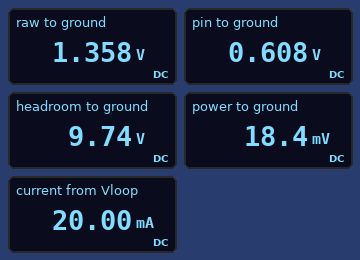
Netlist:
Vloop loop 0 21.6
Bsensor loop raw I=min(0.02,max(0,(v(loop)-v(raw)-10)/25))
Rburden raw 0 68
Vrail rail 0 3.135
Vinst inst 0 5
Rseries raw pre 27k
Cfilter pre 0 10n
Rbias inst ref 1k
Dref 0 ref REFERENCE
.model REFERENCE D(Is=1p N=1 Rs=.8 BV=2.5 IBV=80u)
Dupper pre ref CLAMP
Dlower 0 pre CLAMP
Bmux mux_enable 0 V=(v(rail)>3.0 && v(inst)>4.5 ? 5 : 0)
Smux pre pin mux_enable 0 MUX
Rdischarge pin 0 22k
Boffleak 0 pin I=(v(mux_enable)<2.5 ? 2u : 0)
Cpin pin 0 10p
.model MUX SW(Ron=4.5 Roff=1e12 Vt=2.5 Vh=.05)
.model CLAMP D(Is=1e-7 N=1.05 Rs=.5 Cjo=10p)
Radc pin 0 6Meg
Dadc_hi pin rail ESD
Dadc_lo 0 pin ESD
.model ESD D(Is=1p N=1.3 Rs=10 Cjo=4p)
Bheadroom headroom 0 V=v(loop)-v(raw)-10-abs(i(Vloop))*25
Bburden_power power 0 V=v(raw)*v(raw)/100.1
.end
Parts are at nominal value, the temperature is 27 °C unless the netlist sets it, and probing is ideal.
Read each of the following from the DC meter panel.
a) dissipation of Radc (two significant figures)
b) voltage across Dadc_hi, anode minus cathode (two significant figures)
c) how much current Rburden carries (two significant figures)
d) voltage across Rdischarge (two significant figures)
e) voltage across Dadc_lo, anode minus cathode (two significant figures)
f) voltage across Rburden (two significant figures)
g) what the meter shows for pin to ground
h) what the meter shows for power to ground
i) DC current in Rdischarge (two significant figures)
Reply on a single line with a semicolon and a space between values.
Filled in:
62 nW; -2.5 V; 20 mA; 610 mV; -610 mV; 1.4 V; 0.608 V; 18.4 mV; 28 µA
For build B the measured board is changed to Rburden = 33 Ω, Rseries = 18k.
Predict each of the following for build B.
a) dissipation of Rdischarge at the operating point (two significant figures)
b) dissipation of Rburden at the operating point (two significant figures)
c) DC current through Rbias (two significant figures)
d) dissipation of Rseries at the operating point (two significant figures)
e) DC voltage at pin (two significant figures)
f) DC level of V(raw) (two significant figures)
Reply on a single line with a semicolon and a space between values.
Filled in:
6.0 µW; 13 mW; 2.4 mA; 4.9 µW; 360 mV; 660 mV
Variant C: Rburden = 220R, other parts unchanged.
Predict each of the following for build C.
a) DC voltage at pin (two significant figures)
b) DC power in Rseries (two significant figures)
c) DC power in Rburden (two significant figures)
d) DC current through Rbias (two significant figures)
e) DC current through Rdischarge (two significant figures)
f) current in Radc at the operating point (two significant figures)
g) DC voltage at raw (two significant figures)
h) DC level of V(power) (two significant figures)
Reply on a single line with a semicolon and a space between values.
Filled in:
2.0 V; 220 µW; 87 mW; 2.4 mA; 89 µA; 330 nA; 4.4 V; 190 mV
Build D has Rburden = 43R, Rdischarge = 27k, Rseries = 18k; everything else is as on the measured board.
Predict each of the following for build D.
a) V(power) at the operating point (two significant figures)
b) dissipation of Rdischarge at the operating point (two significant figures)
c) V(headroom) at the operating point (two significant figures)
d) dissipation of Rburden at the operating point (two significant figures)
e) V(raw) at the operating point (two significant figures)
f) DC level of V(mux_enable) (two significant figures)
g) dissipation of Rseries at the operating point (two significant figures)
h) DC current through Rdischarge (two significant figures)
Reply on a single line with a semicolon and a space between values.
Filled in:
7.4 mV; 9.8 µW; 10 V; 17 mW; 860 mV; 5.0 V; 6.6 µW; 19 µA
